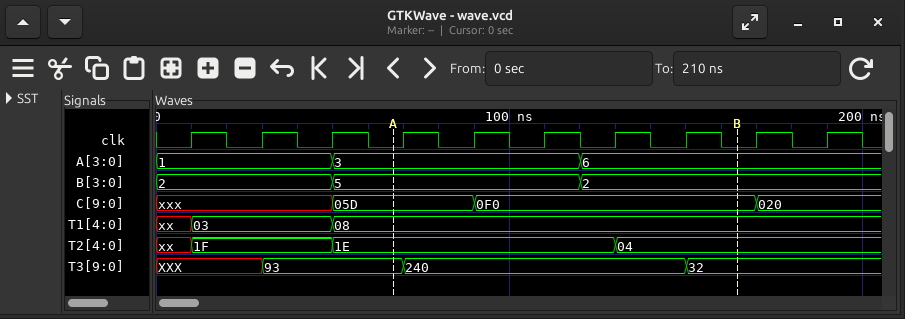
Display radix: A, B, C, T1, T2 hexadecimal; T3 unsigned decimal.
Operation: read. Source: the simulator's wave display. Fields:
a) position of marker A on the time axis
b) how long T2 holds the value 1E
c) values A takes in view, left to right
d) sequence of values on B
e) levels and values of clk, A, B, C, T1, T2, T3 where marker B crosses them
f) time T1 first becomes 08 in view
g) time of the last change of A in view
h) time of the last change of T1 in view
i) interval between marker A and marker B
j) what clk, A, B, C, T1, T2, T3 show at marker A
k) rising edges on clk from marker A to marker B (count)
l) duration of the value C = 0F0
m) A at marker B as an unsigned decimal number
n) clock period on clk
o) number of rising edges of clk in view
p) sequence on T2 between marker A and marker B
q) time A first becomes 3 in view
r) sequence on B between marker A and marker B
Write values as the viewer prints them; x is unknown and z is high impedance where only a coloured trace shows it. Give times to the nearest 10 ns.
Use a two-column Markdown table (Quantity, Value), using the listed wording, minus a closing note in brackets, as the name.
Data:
| Quantity | Value |
|---|---|
| position of marker A on the time axis | 70 ns |
| how long T2 holds the value 1E | 80 ns |
| values A takes in view, left to right | 1, 3, 6 |
| sequence of values on B | 2, 5, 2 |
| levels and values of clk, A, B, C, T1, T2, T3 where marker B crosses them | clk=0, A=6, B=2, C=0F0, T1=08, T2=04, T3=32 |
| time T1 first becomes 08 in view | 50 ns |
| time of the last change of A in view | 120 ns |
| time of the last change of T1 in view | 50 ns |
| interval between marker A and marker B | 100 ns |
| what clk, A, B, C, T1, T2, T3 show at marker A | clk=0, A=3, B=5, C=05D, T1=08, T2=1E, T3=93 |
| rising edges on clk from marker A to marker B | 5 |
| duration of the value C = 0F0 | 80 ns |
| A at marker B as an unsigned decimal number | 6 |
| clock period on clk | 20 ns |
| number of rising edges of clk in view | 10 |
| sequence on T2 between marker A and marker B | 1E, 04 |
| time A first becomes 3 in view | 50 ns |
| sequence on B between marker A and marker B | 5, 2 |
